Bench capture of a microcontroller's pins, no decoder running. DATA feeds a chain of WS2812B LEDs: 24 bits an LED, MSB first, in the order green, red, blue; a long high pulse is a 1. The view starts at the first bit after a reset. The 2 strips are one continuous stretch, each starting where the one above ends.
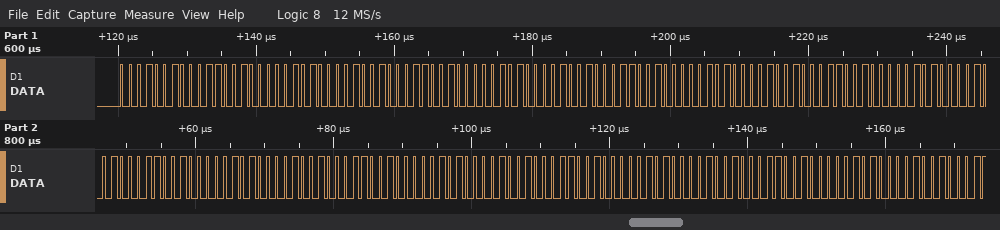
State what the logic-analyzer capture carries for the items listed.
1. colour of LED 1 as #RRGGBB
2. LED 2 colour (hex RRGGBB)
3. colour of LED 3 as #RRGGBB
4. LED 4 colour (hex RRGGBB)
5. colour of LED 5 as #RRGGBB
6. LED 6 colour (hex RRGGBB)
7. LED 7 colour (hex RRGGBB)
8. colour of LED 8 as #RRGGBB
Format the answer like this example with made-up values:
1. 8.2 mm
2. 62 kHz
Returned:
1. #32120A
2. #32120A
3. #32120A
4. #32120A
5. #32120A
6. #32120A
7. #32120A
8. #32120A
